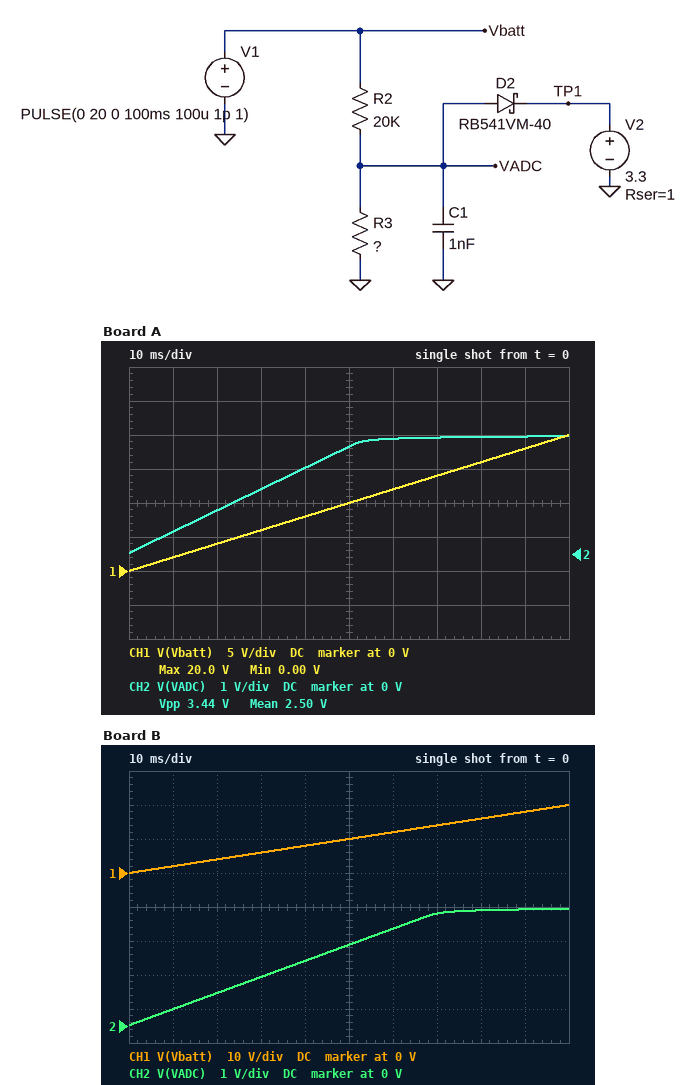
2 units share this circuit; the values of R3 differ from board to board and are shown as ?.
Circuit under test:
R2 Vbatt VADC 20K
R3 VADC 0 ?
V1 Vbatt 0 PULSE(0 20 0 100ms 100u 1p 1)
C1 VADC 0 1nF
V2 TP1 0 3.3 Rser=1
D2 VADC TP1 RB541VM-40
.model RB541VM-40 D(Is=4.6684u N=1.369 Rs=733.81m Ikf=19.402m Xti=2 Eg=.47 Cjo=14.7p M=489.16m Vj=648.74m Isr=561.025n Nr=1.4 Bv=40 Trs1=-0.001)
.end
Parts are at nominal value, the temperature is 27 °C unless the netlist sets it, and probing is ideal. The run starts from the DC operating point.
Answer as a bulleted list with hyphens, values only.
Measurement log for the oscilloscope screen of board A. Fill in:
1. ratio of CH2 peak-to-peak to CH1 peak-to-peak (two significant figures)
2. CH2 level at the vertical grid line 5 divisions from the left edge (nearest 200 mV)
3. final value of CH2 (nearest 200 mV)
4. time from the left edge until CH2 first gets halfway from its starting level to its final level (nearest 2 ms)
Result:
- 0.17
- 3.2 V
- 3.4 V
- 28 ms
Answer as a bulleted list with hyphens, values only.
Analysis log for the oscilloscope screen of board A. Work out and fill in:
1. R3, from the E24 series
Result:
- 9.1 kΩ
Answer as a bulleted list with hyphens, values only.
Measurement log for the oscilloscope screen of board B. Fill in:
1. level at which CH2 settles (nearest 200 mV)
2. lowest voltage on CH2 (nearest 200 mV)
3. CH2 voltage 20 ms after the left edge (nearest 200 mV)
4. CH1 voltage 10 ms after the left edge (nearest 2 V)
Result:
- 3.4 V
- 0 V
- 1.0 V
- 2 V
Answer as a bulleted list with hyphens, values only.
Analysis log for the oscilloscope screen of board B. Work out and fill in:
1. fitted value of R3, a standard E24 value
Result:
- 6.2 kΩ
